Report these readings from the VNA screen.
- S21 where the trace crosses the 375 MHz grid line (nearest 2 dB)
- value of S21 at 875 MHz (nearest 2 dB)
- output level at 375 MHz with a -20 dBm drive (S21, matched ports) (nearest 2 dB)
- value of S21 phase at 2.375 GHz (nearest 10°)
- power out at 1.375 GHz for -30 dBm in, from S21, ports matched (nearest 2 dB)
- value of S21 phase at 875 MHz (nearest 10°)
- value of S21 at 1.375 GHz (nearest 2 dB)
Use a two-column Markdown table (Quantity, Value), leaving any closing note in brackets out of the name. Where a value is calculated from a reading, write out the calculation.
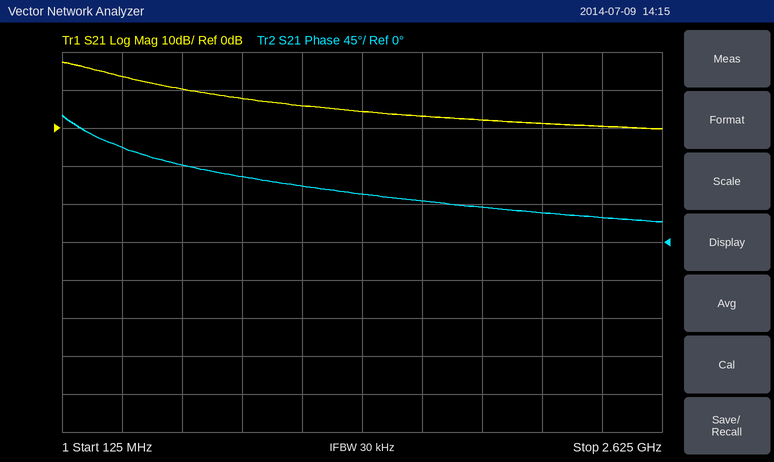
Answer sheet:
| Quantity | Value |
|---|---|
| S21 where the trace crosses the 375 MHz grid line | 14 dB |
| value of S21 at 875 MHz | 8 dB |
| output level at 375 MHz with a -20 dBm drive (S21, matched ports) | -20 dBm + (14 dB) = -6 dBm |
| value of S21 phase at 2.375 GHz | 30° |
| power out at 1.375 GHz for -30 dBm in, from S21, ports matched | -30 dBm + (4 dB) = -26 dBm |
| value of S21 phase at 875 MHz | 80° |
| value of S21 at 1.375 GHz | 4 dB |
